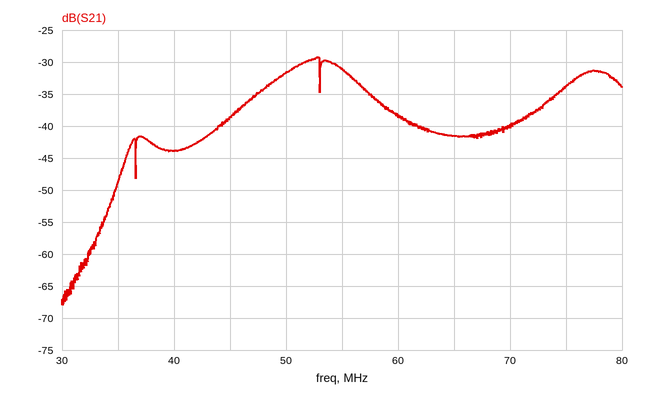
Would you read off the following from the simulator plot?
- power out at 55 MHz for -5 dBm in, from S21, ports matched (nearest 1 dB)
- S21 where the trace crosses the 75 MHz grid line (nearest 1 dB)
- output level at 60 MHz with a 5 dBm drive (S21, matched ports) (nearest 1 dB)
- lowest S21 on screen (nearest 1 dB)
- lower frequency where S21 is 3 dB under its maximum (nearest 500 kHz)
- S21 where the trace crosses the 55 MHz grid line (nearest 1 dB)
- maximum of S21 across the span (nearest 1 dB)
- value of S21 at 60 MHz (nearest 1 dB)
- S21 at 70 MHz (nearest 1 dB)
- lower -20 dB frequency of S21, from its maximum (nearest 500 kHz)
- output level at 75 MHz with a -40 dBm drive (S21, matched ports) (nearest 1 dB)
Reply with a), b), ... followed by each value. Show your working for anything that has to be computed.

a) -5 dBm + (-31 dB) = -36 dBm
b) -34 dB
c) 5 dBm + (-38 dB) = -33 dBm
d) -68 dB
e) 49.5 MHz
f) -31 dB
g) -29 dB
h) -38 dB
i) -40 dB
j) 35.0 MHz
k) -40 dBm + (-34 dB) = -74 dBm
